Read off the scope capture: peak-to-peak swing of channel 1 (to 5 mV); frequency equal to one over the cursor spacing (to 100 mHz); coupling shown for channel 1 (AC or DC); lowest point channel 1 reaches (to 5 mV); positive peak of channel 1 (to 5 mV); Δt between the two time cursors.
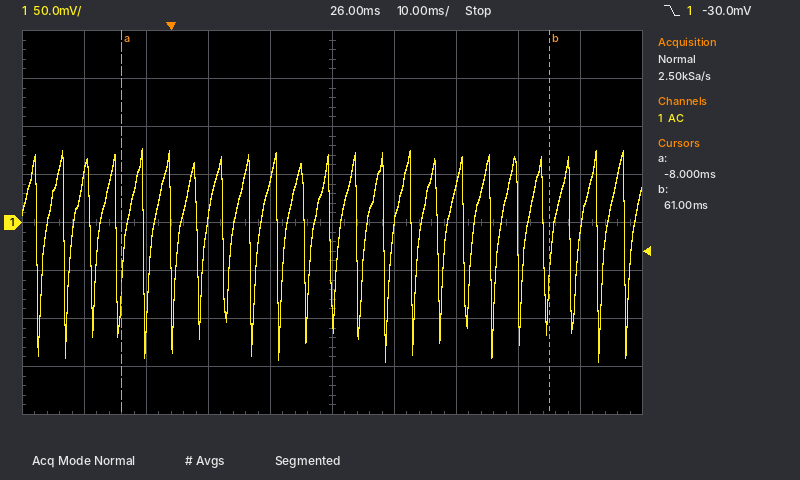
220 mV
14.5 Hz
AC
-145 mV
75 mV
69 ms
